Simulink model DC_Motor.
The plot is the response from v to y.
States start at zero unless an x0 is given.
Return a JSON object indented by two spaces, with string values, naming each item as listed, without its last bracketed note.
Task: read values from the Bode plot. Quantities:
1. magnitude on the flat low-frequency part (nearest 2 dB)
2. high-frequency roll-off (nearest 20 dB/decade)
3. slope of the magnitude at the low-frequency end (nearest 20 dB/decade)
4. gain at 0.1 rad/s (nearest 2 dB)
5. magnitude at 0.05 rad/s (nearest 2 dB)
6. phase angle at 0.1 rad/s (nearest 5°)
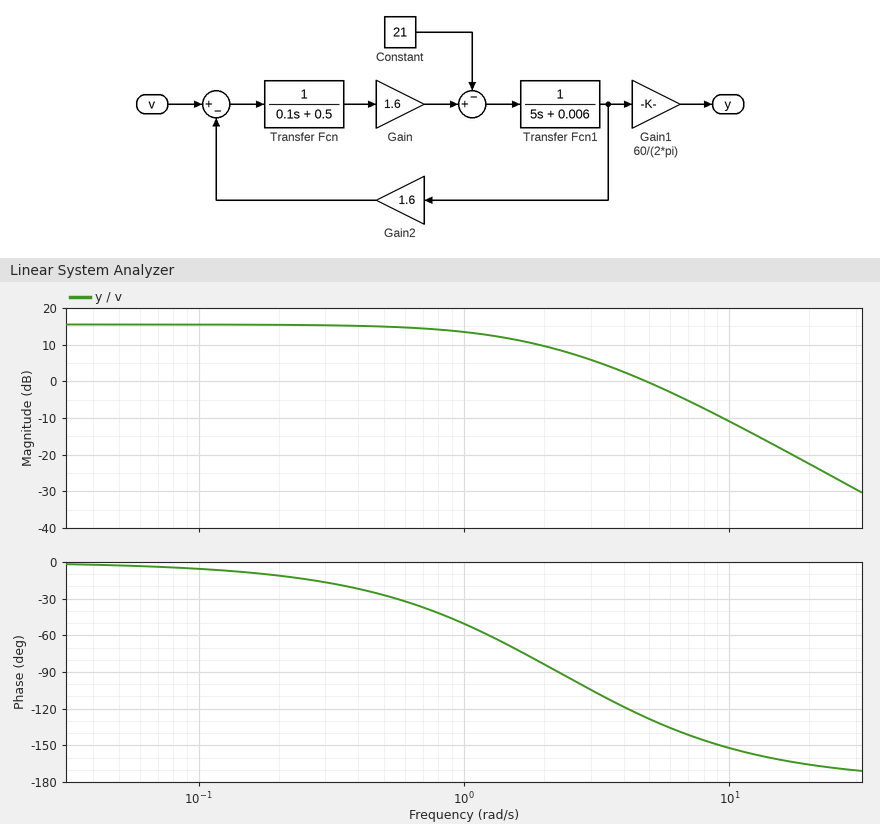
{
  "magnitude on the flat low-frequency part": "16 dB",
  "high-frequency roll-off": "-40 dB/decade",
  "slope of the magnitude at the low-frequency end": "0 dB/decade",
  "gain at 0.1 rad/s": "16 dB",
  "magnitude at 0.05 rad/s": "16 dB",
  "phase angle at 0.1 rad/s": "-5°"
}
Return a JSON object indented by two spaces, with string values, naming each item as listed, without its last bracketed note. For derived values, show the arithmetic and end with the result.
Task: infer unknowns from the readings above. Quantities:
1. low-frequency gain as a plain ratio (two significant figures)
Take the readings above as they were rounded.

{
  "low-frequency gain as a plain ratio": "10^(16 / 20) = 6.3"
}
